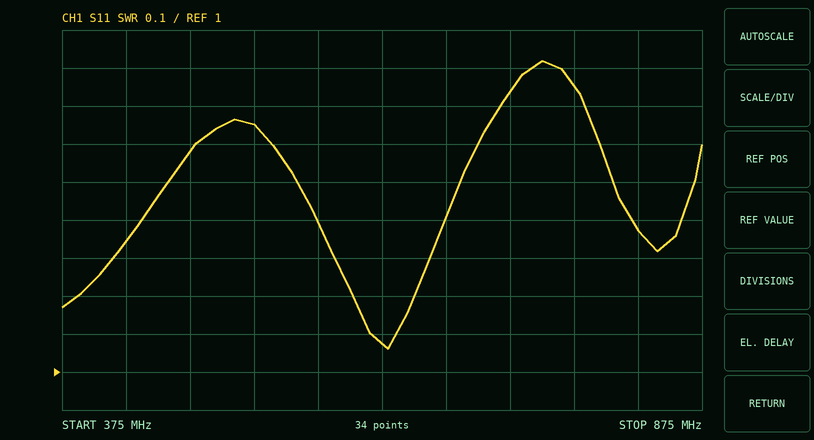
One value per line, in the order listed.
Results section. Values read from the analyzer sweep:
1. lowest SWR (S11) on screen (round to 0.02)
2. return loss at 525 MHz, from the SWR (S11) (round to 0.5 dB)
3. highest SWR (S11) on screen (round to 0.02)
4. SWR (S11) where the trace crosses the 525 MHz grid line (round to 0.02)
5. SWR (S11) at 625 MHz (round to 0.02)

1.06
12.0 dB
1.82
1.66
1.08
